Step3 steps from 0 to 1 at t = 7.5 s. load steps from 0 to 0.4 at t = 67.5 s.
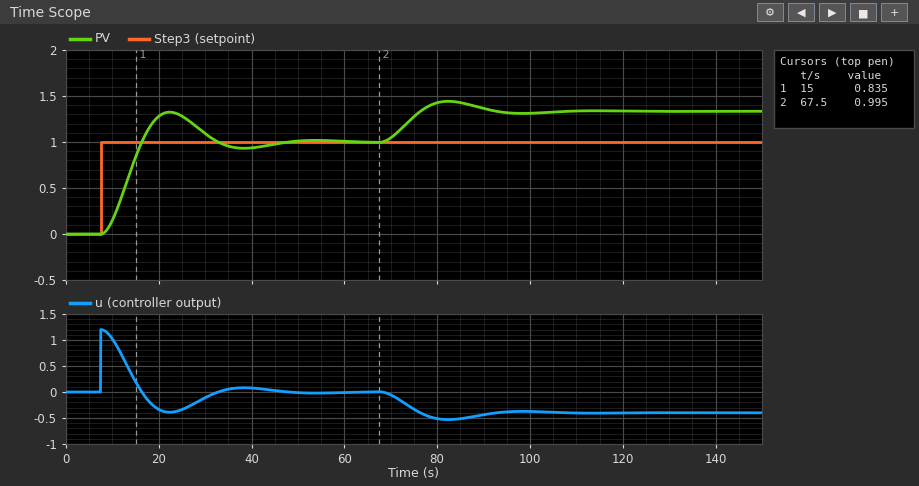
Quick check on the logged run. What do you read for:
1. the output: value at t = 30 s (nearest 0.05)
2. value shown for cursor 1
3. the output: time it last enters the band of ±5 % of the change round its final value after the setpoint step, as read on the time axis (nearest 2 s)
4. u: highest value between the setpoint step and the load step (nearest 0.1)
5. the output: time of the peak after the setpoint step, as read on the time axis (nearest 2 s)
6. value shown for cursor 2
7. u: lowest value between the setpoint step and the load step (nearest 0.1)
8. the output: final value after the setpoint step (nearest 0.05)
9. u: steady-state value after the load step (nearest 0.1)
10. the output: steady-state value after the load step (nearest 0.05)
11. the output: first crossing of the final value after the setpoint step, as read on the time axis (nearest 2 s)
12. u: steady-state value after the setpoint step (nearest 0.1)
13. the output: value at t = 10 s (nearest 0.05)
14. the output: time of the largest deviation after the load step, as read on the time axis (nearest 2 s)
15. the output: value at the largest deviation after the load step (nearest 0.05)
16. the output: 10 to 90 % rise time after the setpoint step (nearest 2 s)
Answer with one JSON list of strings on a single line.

["1.10", "0.835", "42 s", "1.2", "22 s", "0.995", "-0.4", "1.00", "-0.4", "1.35", "16 s", "0.0", "0.15", "82 s", "1.45", "6 s"]
